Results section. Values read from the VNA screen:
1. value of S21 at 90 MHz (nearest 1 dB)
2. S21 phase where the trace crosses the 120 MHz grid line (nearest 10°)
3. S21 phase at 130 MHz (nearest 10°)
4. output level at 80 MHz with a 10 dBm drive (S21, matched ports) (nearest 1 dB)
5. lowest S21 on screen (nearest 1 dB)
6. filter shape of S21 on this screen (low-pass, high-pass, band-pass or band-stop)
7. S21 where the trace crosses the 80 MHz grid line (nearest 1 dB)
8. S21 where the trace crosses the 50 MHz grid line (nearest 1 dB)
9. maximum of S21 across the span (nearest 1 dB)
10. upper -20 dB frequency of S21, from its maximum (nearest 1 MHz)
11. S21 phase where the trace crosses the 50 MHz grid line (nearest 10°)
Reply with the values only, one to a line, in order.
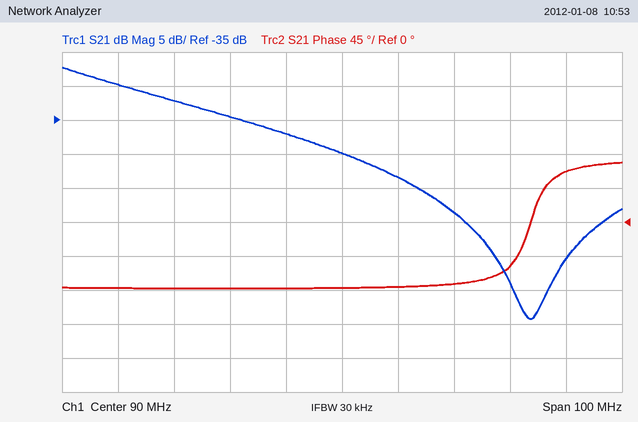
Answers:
-40 dB
-60°
70°
-27 dBm
-64 dB
low-pass
-37 dB
-30 dB
-27 dB
108 MHz
-90°
